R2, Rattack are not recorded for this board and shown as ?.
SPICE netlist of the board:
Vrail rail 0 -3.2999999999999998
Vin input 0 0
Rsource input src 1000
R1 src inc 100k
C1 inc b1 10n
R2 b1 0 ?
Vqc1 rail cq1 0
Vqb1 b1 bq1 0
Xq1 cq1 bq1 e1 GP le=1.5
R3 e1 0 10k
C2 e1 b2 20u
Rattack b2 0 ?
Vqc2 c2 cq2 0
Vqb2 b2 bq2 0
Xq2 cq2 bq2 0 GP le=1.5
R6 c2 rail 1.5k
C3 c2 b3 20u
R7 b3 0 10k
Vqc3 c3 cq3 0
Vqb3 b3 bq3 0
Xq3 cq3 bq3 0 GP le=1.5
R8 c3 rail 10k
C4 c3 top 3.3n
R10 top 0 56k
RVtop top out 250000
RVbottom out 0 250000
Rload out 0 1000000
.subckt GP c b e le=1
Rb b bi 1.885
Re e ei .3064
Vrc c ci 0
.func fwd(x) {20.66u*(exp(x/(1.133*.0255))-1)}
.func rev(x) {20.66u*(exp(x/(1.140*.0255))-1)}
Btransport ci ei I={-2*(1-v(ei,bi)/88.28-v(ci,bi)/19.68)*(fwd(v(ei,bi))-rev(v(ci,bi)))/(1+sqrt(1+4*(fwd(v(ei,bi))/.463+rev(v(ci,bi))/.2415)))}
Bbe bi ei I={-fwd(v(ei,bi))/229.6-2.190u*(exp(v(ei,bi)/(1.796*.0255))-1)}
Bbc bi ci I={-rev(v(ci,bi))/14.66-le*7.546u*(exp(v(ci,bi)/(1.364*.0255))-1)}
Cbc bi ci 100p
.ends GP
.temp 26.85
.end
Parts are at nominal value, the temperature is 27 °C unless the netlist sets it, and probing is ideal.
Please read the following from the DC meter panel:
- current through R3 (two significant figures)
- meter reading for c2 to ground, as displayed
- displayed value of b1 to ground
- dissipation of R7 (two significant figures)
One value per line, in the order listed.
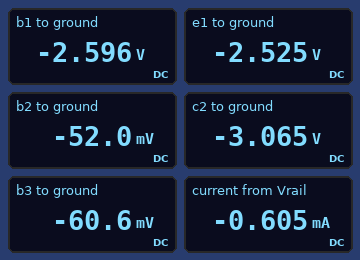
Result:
250 µA
-3.065 V
-2.596 V
370 nW
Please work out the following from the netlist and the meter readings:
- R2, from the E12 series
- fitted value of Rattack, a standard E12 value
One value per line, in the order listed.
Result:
680 kΩ
6.8 kΩ
